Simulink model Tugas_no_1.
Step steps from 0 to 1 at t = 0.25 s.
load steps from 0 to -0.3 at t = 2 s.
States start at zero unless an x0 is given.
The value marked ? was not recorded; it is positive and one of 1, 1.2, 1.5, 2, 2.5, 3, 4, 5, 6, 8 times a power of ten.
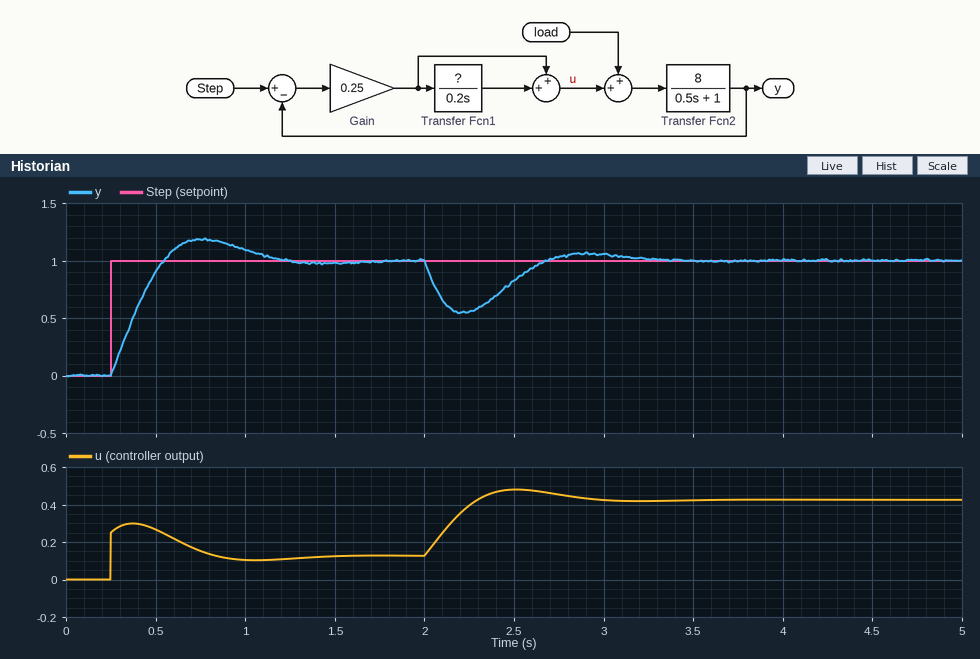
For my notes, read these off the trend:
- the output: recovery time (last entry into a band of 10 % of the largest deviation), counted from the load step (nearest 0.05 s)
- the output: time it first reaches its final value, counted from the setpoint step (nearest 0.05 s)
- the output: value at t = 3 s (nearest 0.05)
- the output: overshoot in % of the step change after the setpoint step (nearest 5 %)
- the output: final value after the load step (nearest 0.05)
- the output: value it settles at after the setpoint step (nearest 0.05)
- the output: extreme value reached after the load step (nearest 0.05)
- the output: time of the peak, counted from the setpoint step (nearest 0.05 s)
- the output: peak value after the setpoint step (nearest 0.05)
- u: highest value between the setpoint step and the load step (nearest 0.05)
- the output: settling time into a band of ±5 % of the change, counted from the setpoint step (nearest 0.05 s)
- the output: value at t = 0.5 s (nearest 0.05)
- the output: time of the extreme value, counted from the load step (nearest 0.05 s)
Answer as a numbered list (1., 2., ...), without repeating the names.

1. 1.05 s
2. 0.30 s
3. 1.05
4. 20 %
5. 1.00
6. 1.00
7. 0.55
8. 0.50 s
9. 1.20
10. 0.30
11. 0.85 s
12. 0.90
13. 0.20 s
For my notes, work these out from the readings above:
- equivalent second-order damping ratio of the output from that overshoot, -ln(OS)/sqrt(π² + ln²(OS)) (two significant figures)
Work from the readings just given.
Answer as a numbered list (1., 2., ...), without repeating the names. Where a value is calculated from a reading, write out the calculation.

1. ln(0.2) = -1.609; 1.609 / sqrt(9.870 + 2.590) = 0.46
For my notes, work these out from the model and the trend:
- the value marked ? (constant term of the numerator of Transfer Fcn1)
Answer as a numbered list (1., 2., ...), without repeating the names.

1. 1.5
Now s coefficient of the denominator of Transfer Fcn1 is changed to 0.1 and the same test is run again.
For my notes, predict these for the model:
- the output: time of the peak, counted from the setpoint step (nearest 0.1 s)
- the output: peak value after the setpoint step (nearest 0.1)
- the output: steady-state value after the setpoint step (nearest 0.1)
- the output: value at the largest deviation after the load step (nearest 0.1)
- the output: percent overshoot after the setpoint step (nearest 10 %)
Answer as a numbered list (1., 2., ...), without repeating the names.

1. 0.4 s
2. 1.3
3. 1.0
4. 0.6
5. 30 %
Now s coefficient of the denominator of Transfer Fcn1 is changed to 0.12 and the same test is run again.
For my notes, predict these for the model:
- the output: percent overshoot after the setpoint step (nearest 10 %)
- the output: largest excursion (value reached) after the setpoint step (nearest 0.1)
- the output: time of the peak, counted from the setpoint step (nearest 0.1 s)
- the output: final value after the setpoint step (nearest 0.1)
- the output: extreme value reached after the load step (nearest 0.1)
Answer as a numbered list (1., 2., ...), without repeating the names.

1. 30 %
2. 1.3
3. 0.4 s
4. 1.0
5. 0.6
